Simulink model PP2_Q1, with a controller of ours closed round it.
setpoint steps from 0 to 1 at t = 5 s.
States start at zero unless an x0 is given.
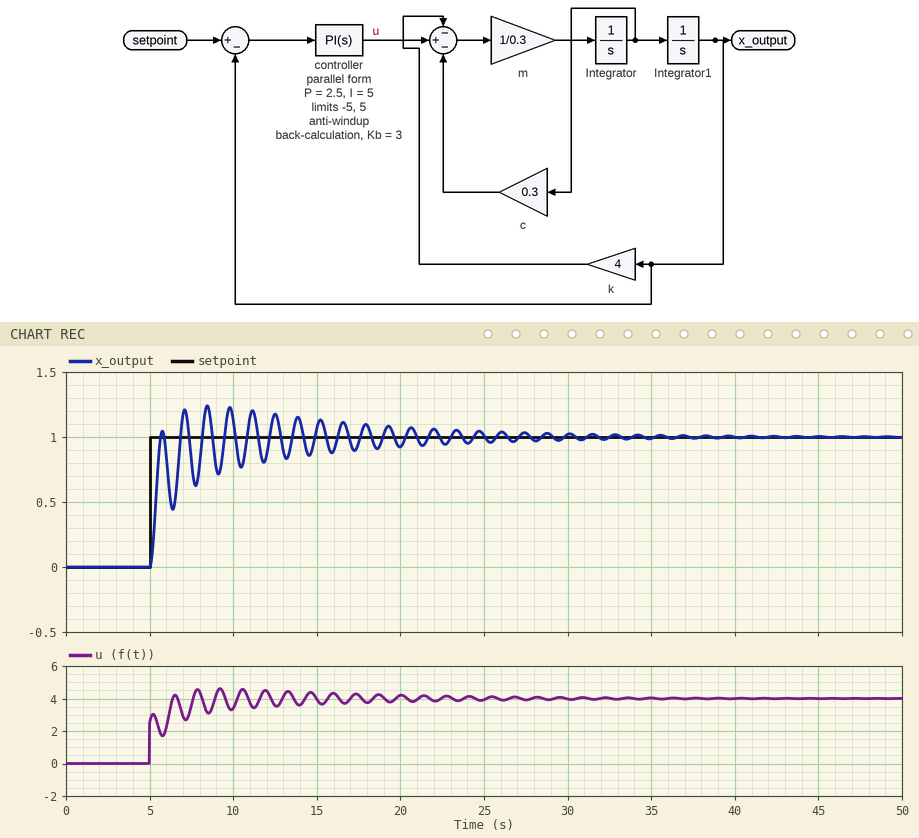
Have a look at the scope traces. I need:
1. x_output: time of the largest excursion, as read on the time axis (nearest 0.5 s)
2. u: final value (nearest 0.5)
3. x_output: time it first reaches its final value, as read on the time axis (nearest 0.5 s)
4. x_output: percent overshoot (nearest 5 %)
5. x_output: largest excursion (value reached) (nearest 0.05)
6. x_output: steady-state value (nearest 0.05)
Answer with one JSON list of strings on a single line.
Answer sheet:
["8.5 s", "4.0", "5.5 s", "25 %", "1.25", "1.00"]
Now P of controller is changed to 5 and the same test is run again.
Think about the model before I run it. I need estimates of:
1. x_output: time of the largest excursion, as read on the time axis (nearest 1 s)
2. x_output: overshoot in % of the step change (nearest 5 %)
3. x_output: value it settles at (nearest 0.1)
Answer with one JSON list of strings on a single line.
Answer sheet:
["7 s", "20 %", "1.0"]
